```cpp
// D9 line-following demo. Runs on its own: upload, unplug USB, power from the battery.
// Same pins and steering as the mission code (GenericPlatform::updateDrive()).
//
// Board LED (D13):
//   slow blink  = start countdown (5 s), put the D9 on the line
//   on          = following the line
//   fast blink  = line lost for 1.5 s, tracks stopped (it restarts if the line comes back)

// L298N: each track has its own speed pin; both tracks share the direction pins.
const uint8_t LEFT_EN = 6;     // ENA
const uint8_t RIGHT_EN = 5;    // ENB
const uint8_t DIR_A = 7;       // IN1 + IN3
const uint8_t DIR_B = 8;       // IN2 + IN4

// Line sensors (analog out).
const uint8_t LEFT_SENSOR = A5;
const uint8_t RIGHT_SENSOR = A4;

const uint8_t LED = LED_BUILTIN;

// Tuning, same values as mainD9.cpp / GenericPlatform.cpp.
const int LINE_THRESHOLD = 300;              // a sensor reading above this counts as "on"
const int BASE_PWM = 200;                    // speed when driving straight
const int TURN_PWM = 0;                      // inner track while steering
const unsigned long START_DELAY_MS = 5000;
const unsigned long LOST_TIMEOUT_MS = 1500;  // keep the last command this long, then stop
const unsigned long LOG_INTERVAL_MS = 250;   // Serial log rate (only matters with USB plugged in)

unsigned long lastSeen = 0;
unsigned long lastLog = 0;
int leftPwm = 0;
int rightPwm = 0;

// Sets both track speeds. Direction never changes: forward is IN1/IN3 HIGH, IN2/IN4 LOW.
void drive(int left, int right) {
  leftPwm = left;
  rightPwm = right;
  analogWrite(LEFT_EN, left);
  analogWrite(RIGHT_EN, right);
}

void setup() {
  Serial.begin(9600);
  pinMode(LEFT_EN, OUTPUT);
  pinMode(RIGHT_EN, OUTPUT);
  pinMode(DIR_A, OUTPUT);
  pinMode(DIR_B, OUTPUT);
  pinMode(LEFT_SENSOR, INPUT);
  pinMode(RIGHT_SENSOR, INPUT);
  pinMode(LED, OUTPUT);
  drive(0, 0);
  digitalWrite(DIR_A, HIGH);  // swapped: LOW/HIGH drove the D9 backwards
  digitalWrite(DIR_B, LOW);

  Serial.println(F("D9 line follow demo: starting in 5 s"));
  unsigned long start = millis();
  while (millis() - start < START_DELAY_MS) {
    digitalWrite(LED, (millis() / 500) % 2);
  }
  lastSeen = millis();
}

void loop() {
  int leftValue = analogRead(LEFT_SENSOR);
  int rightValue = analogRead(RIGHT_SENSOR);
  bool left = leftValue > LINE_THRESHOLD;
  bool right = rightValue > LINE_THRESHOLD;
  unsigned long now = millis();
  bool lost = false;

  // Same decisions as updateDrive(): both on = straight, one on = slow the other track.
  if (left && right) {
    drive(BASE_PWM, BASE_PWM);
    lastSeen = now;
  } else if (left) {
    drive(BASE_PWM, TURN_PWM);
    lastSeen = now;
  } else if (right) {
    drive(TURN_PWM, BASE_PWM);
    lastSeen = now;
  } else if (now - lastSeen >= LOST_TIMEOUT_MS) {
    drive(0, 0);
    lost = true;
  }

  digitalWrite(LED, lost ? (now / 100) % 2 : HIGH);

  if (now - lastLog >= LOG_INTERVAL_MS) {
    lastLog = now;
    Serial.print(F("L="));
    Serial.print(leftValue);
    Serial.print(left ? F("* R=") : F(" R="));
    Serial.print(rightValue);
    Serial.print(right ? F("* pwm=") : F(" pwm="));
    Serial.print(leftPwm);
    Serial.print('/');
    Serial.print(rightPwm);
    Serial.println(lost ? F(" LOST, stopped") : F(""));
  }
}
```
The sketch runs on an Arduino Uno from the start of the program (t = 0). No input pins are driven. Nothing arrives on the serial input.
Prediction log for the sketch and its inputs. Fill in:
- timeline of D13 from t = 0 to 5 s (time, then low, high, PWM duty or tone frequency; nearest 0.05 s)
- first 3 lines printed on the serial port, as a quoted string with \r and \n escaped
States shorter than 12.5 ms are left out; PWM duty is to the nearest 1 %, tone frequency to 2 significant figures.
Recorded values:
0 s low; 0.5 s high; 1 s low; 1.5 s high; 2 s low; 2.5 s high; 3 s low; 3.5 s high; 4 s low; 4.5 s high
"D9 line follow demo: starting in 5 s\r\nL=0 R=0 pwm=0/0\r\nL=0 R=0 pwm=0/0\r\n"
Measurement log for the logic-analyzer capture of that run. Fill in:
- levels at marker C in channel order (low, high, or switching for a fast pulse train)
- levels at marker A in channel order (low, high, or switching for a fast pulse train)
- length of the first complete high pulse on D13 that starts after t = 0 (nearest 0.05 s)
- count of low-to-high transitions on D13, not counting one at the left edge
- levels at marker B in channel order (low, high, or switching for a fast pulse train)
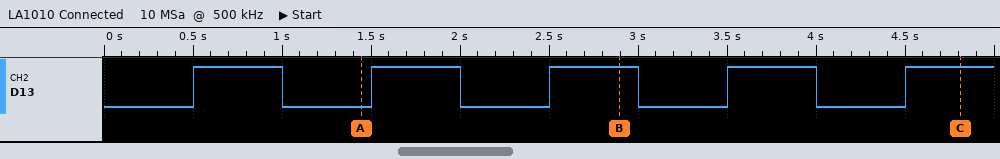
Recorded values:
D13 high
D13 low
0.50 s
5
D13 high
